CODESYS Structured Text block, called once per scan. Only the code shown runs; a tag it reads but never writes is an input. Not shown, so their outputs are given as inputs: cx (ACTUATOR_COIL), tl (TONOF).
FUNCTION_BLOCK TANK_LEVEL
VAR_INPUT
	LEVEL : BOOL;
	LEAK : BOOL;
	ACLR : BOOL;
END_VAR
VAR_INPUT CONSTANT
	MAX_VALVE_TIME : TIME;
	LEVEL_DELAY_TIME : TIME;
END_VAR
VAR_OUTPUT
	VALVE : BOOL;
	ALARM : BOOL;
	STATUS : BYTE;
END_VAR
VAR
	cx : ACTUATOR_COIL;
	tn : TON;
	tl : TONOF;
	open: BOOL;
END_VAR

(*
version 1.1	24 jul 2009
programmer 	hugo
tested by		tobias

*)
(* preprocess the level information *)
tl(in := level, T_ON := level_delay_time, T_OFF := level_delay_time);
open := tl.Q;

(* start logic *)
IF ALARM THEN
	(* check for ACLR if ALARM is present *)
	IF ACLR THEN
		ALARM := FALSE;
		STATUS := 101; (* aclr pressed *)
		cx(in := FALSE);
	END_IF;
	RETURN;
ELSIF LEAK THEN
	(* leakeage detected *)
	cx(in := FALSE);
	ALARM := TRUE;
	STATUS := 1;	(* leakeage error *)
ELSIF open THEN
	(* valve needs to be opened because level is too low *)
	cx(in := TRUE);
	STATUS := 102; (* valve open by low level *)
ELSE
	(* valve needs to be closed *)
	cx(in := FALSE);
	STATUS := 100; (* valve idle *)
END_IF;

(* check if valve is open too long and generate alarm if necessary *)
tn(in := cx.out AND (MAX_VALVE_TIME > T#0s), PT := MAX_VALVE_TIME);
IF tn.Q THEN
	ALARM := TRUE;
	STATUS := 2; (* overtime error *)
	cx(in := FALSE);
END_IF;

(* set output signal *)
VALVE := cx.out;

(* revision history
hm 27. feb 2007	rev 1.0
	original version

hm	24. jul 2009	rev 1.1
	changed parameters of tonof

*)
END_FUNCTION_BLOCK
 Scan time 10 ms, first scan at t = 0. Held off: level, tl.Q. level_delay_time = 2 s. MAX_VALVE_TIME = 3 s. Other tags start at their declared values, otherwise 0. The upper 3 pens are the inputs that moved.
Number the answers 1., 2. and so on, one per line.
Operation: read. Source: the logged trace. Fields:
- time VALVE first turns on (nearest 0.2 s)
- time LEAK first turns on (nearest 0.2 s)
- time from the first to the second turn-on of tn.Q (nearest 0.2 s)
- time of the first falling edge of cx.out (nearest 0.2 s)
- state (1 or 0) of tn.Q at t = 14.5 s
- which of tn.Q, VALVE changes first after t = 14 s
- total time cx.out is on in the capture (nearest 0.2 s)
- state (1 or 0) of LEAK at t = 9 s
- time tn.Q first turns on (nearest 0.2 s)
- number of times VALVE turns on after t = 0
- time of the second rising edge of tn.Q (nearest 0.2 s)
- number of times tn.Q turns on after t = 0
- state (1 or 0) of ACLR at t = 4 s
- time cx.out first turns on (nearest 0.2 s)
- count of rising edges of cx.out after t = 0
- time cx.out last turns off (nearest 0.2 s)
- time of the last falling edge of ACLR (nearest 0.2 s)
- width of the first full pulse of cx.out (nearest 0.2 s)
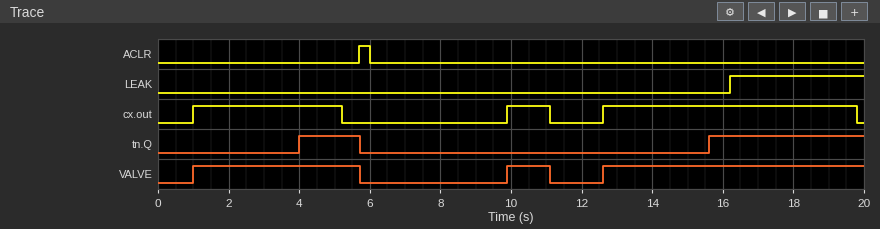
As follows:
1. 1.0 s
2. 16.2 s
3. 11.6 s
4. 5.2 s
5. 0
6. tn.Q
7. 12.6 s
8. 0
9. 4.0 s
10. 3
11. 15.6 s
12. 2
13. 0
14. 1.0 s
15. 3
16. 19.8 s
17. 6.0 s
18. 4.2 s
